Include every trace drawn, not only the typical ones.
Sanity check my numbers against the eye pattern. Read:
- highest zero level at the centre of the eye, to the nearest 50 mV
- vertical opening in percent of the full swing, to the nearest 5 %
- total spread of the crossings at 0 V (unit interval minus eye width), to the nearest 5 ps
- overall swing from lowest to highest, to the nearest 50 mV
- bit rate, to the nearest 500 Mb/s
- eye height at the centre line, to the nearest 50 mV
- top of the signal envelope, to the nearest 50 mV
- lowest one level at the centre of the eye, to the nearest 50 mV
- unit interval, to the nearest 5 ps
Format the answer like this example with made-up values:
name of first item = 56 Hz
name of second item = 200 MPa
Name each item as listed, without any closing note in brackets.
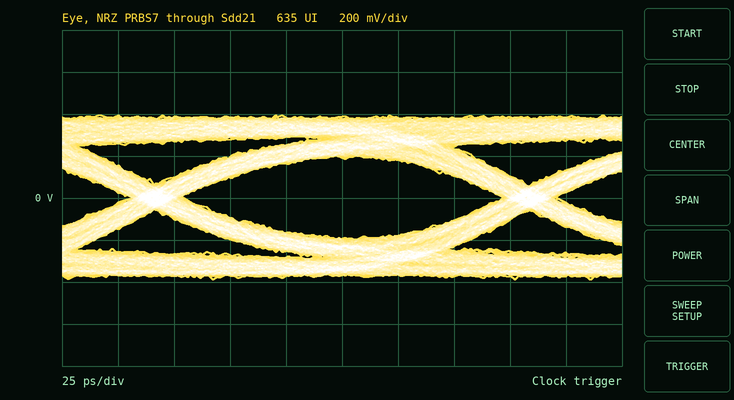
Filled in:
highest zero level at the centre of the eye, to the nearest 50 mV = -200 mV
vertical opening in percent of the full swing, to the nearest 5 % = 50 %
total spread of the crossings at 0 V (unit interval minus eye width), to the nearest 5 ps = 25 ps
overall swing from lowest to highest, to the nearest 50 mV = 800 mV
bit rate, to the nearest 500 Mb/s = 6.0 Gb/s
eye height at the centre line, to the nearest 50 mV = 400 mV
top of the signal envelope, to the nearest 50 mV = 400 mV
lowest one level at the centre of the eye, to the nearest 50 mV = 200 mV
unit interval, to the nearest 5 ps = 165 ps
